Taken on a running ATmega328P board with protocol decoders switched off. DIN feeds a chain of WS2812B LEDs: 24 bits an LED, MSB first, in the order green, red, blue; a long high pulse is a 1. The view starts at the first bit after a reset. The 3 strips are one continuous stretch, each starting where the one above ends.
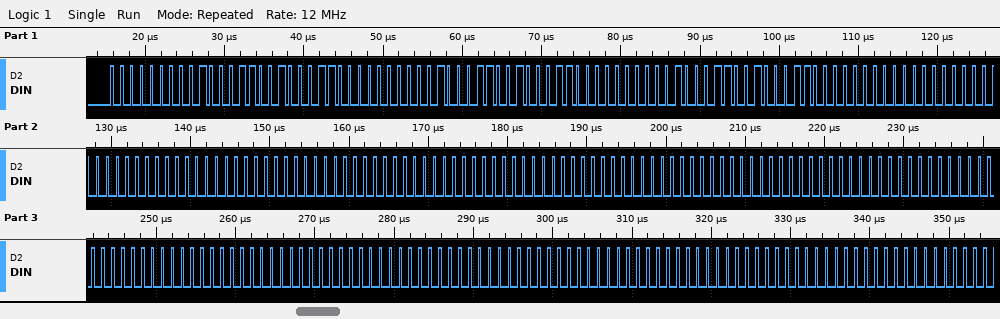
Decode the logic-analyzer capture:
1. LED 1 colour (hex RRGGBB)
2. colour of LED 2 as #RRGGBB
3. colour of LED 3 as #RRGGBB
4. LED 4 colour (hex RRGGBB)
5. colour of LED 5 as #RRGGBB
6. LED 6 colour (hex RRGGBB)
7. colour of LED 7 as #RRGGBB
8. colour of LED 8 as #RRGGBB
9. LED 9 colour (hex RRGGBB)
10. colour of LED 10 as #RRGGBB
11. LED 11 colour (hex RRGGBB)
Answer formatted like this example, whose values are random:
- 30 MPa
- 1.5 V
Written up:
- #460046
- #460046
- #460046
- #000000
- #000000
- #000000
- #000000
- #000000
- #000000
- #000000
- #000000
